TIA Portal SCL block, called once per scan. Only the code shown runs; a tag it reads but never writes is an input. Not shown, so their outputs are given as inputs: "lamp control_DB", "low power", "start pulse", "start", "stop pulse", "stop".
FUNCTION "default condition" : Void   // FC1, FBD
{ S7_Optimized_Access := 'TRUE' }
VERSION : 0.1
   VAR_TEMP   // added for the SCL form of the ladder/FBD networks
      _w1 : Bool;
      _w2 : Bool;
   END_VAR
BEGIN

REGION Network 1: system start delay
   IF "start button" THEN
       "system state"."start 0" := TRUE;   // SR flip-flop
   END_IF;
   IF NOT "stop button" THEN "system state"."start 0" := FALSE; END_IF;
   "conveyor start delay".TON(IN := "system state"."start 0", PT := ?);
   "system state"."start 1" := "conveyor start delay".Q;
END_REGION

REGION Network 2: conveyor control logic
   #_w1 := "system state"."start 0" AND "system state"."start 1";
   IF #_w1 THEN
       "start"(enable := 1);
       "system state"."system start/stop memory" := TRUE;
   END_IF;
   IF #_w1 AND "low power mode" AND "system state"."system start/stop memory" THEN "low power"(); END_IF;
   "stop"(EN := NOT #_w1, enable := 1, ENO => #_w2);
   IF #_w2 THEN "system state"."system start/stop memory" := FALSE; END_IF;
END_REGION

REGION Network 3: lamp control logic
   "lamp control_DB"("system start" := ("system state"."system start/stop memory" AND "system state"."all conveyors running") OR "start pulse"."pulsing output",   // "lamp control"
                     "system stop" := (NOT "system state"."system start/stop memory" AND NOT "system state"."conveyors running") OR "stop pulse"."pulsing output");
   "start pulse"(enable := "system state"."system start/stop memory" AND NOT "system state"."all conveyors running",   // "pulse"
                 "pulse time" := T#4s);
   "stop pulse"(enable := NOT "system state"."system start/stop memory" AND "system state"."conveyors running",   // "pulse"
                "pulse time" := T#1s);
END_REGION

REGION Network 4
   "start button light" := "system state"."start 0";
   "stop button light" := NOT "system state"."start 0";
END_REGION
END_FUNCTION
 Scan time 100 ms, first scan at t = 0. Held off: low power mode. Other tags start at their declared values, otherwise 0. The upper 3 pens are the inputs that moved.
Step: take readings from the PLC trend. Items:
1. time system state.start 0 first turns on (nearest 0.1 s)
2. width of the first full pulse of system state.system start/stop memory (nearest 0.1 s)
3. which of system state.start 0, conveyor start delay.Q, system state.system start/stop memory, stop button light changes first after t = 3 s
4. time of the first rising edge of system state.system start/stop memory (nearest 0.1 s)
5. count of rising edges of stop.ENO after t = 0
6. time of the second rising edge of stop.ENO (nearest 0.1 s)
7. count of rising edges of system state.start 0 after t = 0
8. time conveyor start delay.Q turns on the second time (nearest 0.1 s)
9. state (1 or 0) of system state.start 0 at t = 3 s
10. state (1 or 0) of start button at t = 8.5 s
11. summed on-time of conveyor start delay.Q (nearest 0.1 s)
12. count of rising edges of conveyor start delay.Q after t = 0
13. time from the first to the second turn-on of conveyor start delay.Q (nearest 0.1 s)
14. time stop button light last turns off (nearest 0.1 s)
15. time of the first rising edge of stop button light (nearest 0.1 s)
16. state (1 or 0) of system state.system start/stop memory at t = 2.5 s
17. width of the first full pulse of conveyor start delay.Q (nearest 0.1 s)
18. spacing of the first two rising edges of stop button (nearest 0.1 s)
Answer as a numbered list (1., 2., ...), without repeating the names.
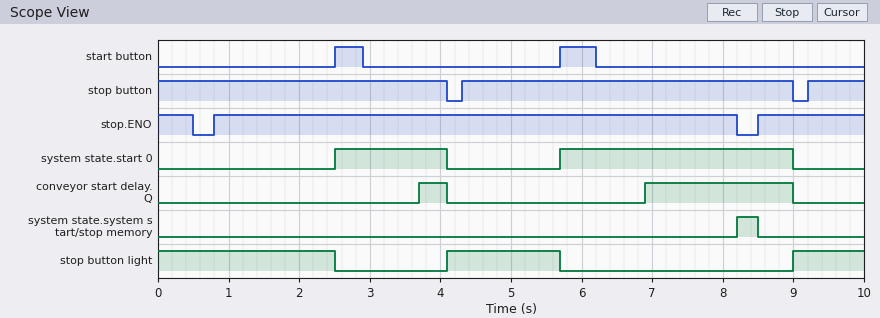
1. 2.5 s
2. 0.3 s
3. conveyor start delay.Q
4. 8.2 s
5. 2
6. 8.5 s
7. 2
8. 6.9 s
9. 1
10. 0
11. 2.5 s
12. 2
13. 3.2 s
14. 5.7 s
15. 4.1 s
16. 0
17. 0.4 s
18. 4.9 s
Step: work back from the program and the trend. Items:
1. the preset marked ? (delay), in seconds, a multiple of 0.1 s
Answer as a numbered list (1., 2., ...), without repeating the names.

1. 1.2 s
